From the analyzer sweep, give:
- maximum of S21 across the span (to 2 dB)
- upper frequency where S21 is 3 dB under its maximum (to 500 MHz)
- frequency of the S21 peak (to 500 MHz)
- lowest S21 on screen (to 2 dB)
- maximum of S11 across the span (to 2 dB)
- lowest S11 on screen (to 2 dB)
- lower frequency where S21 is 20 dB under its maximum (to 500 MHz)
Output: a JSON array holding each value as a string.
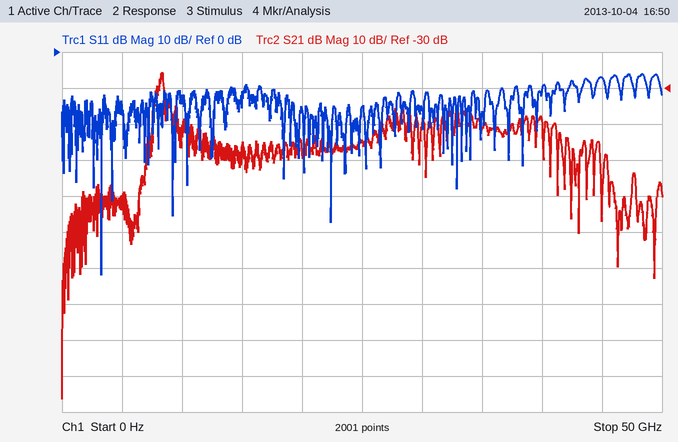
["-26 dB", "8.5 GHz", "8.5 GHz", "-116 dB", "-6 dB", "-62 dB", "7.5 GHz"]
